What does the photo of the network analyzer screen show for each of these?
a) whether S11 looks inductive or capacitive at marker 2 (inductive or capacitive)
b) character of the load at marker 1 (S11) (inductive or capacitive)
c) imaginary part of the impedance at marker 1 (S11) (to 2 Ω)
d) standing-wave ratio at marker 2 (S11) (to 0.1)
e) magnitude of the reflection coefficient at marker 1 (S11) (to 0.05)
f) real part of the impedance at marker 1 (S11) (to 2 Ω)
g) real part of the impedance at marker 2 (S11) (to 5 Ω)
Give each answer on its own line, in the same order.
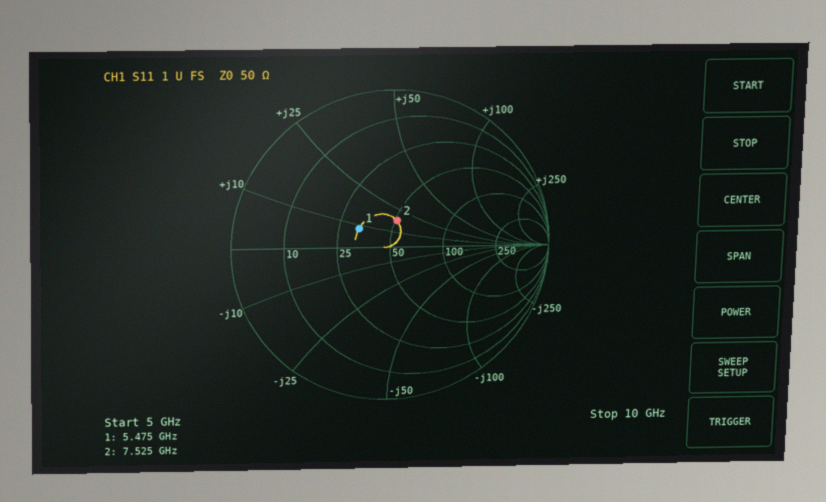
inductive
inductive
+8 Ω
1.4
0.25
32 Ω
50 Ω
